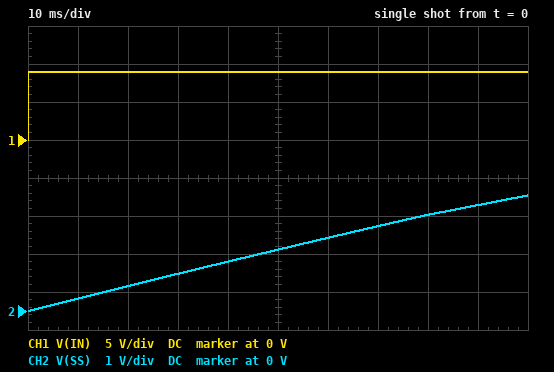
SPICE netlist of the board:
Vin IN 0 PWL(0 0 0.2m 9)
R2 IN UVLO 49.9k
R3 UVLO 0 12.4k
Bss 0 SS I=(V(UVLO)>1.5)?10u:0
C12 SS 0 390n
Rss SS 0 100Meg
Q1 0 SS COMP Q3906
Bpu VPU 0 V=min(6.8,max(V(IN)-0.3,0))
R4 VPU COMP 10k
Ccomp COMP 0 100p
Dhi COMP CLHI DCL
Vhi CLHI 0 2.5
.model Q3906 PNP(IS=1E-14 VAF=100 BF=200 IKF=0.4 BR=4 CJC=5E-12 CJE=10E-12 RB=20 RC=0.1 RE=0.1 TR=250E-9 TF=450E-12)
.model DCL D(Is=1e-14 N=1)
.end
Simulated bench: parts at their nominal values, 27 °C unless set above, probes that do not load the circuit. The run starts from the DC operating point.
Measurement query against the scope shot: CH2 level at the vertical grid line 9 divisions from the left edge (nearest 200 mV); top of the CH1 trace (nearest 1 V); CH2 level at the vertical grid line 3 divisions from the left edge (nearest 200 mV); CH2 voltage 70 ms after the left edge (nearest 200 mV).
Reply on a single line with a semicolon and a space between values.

2.8 V; 9 V; 1.0 V; 2.2 V
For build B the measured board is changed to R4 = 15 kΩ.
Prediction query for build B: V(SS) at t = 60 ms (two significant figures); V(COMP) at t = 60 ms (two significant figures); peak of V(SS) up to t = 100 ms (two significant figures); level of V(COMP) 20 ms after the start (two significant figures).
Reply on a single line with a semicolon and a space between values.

1.8 V; 2.4 V; 2.9 V; 1.2 V
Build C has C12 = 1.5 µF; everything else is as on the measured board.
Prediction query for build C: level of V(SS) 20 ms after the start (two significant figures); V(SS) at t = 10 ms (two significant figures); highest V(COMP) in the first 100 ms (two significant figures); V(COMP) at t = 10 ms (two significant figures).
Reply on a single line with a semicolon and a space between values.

170 mV; 86 mV; 1.5 V; 730 mV
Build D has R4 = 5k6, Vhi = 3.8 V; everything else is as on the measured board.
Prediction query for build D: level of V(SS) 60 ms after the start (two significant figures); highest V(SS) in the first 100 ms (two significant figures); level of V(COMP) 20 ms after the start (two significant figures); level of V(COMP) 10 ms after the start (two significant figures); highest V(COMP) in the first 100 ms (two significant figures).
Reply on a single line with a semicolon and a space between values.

2.2 V; 3.5 V; 1.4 V; 1.0 V; 4.2 V
